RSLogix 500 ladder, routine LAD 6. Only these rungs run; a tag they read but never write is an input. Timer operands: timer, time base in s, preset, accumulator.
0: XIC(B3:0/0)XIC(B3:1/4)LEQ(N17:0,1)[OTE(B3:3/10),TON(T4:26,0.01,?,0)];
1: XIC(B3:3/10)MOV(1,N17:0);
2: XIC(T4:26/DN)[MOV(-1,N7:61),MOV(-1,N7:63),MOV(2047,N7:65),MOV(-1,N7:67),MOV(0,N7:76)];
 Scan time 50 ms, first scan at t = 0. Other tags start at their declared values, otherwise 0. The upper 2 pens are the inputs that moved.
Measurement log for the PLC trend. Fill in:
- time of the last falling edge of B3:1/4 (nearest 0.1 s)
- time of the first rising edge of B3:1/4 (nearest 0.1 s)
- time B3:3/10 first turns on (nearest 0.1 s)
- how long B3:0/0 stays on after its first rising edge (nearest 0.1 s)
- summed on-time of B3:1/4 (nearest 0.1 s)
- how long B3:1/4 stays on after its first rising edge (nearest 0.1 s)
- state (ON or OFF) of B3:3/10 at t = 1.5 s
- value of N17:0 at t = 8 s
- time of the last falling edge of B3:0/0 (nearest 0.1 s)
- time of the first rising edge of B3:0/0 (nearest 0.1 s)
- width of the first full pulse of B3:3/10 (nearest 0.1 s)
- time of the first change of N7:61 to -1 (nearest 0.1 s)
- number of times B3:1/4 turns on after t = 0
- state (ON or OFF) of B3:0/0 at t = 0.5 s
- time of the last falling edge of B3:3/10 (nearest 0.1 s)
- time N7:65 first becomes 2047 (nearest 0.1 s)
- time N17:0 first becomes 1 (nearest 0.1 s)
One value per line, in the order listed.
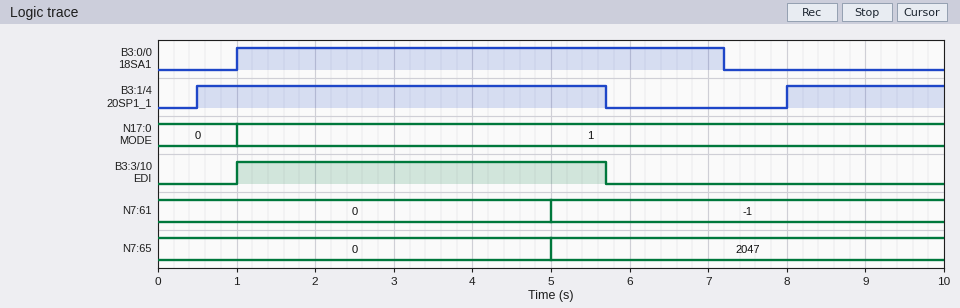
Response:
5.7 s
0.5 s
1.0 s
6.2 s
7.2 s
5.2 s
ON
1
7.2 s
1.0 s
4.7 s
5.0 s
2
OFF
5.7 s
5.0 s
1.0 s
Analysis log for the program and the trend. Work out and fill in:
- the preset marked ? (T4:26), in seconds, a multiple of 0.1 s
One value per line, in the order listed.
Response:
4.0 s
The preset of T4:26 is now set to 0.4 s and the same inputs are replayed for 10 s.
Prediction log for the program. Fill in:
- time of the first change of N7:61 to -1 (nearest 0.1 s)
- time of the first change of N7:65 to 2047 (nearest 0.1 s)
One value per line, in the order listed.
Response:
1.4 s
1.4 s
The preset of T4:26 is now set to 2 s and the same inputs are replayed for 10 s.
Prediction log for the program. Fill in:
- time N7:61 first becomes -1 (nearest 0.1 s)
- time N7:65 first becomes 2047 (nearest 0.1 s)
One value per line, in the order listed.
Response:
3.0 s
3.0 s
